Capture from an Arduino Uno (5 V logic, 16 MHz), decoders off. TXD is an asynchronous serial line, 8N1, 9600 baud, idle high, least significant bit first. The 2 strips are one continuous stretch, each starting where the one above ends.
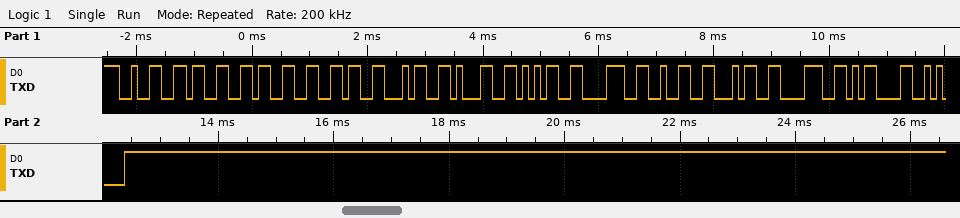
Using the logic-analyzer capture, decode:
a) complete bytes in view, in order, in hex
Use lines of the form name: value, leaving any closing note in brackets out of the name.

complete bytes in view, in order, in hex: 0x32 0x33 0x33 0x36 0x34 0x31 0x35 0x38 0x32 0x34 0x38 0x0D 0x0A
